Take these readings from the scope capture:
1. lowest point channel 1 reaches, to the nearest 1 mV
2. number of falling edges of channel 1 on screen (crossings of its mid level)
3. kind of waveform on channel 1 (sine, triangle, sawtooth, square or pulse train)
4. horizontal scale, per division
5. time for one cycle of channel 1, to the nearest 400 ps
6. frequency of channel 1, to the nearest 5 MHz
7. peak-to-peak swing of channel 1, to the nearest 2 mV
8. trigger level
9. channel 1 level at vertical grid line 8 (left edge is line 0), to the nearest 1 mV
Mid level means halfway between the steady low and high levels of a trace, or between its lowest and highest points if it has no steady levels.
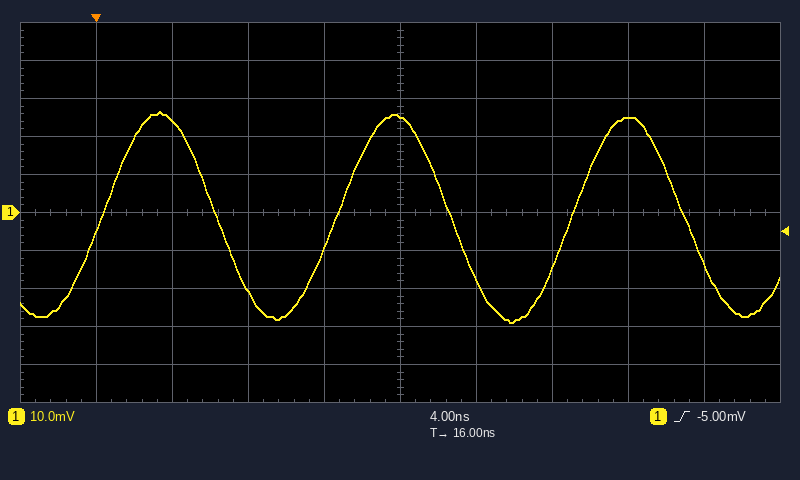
-29 mV
3
sine
4 ns
12.4 ns
80 MHz
56 mV
-5.00 mV
25 mV
